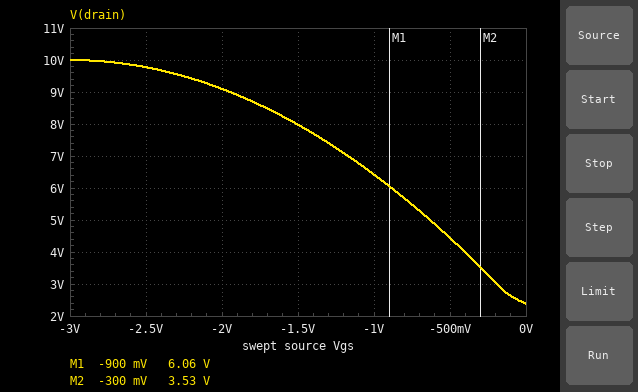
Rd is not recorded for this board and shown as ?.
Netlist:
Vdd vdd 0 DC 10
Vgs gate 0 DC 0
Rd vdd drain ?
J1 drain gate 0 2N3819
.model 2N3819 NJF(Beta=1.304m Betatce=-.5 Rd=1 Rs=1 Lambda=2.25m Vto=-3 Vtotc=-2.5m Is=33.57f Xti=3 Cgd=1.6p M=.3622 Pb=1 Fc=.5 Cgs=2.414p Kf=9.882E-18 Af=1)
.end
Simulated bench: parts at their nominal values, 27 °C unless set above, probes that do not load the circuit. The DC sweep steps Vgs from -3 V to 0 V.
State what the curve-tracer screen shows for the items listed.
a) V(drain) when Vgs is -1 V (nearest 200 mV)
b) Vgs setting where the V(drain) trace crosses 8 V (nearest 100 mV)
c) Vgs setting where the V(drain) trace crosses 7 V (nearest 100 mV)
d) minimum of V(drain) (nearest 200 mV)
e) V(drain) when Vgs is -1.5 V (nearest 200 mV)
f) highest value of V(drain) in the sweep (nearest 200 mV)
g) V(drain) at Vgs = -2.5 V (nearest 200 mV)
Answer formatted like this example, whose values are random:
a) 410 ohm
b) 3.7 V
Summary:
a) 6.4 V
b) -1.5 V
c) -1.2 V
d) 2.4 V
e) 8.0 V
f) 10.0 V
g) 9.8 V
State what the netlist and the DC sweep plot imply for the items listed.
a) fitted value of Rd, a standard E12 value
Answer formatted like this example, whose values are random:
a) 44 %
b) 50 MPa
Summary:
a) 680 Ω
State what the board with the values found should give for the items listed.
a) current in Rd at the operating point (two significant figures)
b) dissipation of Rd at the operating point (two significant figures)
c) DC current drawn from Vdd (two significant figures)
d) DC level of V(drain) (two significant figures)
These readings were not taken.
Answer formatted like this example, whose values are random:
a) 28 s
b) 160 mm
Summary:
a) 11 mA
b) 85 mW
c) 11 mA
d) 2.4 V
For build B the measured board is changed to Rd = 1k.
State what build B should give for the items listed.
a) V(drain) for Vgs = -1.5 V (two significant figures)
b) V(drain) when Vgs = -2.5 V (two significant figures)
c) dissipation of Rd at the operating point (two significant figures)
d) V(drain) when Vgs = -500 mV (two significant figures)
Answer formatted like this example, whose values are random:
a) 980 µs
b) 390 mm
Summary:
a) 7.0 V
b) 9.7 V
c) 73 mW
d) 2.1 V
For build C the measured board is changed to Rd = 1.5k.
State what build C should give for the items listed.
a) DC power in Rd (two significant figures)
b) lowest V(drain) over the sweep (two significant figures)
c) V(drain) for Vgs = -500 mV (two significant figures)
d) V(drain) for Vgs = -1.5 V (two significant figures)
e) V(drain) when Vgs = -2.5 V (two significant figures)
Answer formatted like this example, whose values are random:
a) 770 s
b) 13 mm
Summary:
a) 55 mW
b) 920 mV
c) 1.2 V
d) 5.6 V
e) 9.5 V
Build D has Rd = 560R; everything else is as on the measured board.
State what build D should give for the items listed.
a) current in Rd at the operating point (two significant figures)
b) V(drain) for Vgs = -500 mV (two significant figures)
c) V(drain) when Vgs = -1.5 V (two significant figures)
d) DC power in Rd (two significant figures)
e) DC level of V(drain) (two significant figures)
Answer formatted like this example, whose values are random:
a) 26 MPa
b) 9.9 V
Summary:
a) 12 mA
b) 5.4 V
c) 8.3 V
d) 77 mW
e) 3.4 V
